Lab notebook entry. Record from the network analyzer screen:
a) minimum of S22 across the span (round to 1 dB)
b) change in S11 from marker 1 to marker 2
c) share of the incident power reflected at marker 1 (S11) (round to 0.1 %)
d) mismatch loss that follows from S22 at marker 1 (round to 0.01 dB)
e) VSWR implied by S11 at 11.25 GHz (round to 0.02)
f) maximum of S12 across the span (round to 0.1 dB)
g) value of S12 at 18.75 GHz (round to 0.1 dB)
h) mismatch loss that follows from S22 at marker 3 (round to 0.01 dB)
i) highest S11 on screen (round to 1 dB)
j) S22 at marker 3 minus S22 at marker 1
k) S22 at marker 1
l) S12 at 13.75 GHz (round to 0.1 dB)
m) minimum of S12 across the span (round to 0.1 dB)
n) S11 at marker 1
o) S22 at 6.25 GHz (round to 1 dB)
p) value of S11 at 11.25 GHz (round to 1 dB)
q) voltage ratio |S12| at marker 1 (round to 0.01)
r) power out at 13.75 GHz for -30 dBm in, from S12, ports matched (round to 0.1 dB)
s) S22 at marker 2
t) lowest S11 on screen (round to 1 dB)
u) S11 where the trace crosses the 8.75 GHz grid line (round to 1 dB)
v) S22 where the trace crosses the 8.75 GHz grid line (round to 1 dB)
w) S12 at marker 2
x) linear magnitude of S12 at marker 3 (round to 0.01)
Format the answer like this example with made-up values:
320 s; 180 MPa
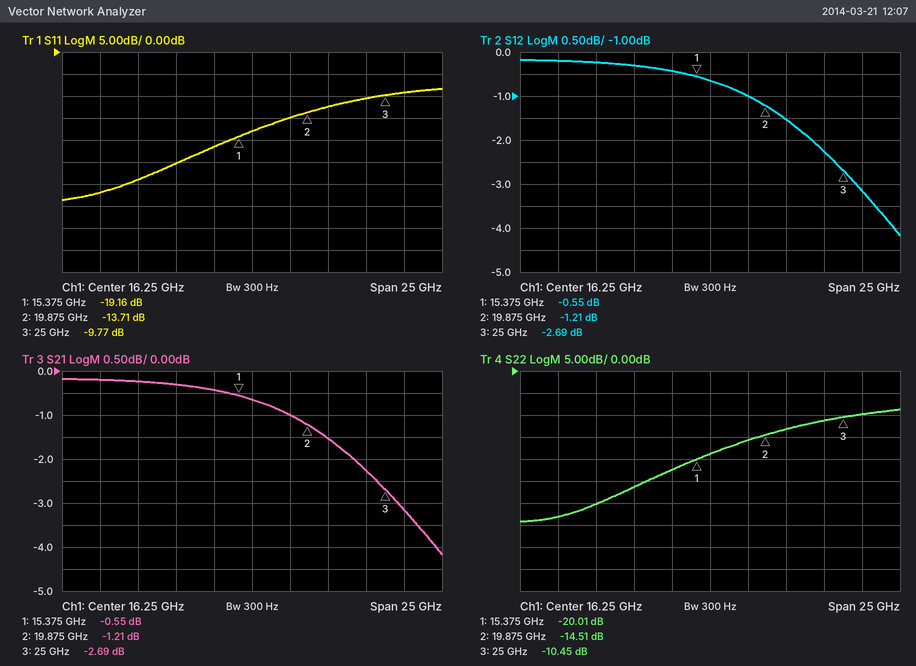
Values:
-34 dB; 5.45 dB; 1.2 %; 0.04 dB; 1.12; -0.2 dB; -1.0 dB; 0.41 dB; -8 dB; 9.56 dB; -20.01 dB; -0.4 dB; -4.2 dB; -19.16 dB; -33 dB; -25 dB; 0.94; -30.4 dBm; -14.51 dB; -34 dB; -29 dB; -30 dB; -1.21 dB; 0.73
